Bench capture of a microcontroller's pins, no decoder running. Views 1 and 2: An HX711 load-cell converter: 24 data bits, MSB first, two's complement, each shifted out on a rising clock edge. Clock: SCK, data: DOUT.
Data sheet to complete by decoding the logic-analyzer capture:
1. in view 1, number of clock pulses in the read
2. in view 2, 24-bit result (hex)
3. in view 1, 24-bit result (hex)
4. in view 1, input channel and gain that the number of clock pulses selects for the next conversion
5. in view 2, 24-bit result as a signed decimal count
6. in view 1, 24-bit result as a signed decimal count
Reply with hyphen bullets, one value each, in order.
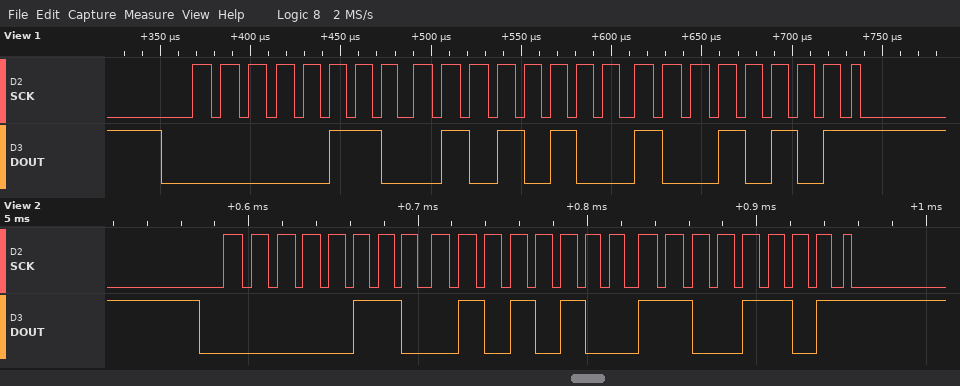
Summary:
- 25
- 0x0654CD
- 0x065495
- channel A, gain 128
- 414925
- 414869
